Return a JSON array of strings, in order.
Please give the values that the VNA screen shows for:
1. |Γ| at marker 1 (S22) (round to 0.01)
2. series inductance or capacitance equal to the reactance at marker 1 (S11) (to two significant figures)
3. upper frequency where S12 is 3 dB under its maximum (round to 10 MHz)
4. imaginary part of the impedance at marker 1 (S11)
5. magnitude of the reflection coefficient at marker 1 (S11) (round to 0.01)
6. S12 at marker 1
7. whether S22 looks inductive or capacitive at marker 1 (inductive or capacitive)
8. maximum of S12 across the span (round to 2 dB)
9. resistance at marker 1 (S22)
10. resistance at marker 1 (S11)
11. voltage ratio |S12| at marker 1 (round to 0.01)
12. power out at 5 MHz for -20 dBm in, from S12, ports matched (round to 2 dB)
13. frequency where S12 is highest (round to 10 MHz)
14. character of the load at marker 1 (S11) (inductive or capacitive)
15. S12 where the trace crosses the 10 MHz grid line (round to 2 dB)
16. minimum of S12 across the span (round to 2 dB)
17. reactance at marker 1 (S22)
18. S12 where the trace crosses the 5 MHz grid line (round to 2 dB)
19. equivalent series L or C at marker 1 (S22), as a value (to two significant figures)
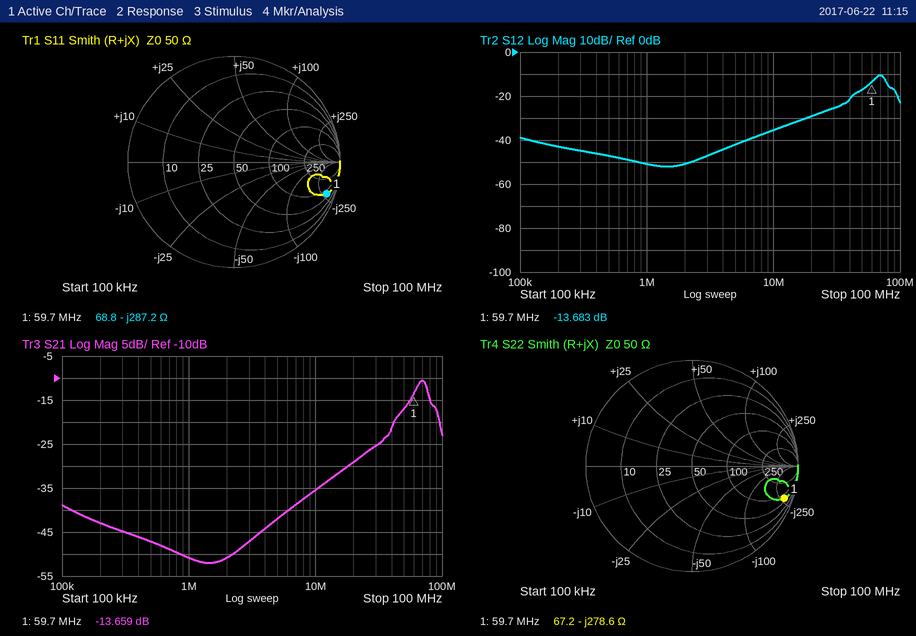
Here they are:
["0.92", "9.3 pF", "80 MHz", "-287.2 Ω", "0.93", "-13.683 dB", "capacitive", "-10 dB", "67.2 Ω", "68.8 Ω", "0.21", "-62 dBm", "70 MHz", "capacitive", "-36 dB", "-52 dB", "-278.6 Ω", "-42 dB", "9.6 pF"]
